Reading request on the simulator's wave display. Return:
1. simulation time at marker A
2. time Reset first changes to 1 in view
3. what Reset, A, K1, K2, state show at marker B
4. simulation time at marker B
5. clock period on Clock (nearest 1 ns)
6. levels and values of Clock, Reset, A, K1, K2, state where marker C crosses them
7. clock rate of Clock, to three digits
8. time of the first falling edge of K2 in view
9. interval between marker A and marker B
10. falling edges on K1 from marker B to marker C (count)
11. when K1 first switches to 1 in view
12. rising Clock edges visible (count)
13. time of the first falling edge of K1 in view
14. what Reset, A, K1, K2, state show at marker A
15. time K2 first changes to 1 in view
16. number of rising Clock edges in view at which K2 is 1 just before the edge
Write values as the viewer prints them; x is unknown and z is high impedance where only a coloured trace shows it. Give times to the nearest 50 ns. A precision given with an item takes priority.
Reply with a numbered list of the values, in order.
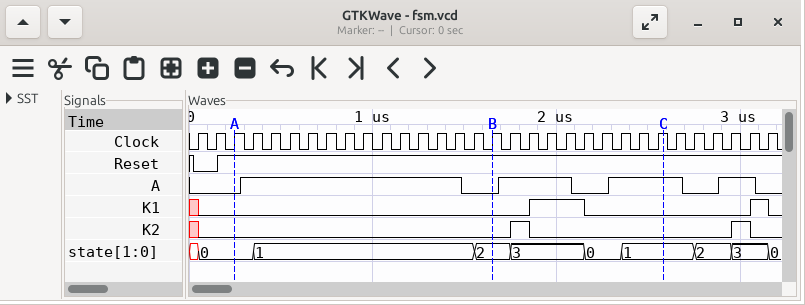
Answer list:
1. 250 ns
2. 150 ns
3. Reset=1, A=0, K1=0, K2=0, state=2
4. 1650 ns
5. 100 ns
6. Clock=1, Reset=1, A=1, K1=0, K2=0, state=1
7. 10.0 MHz
8. 1850 ns
9. 1400 ns
10. 1
11. 1850 ns
12. 32
13. 2150 ns
14. Reset=1, A=0, K1=0, K2=0, state=0
15. 1750 ns
16. 2
